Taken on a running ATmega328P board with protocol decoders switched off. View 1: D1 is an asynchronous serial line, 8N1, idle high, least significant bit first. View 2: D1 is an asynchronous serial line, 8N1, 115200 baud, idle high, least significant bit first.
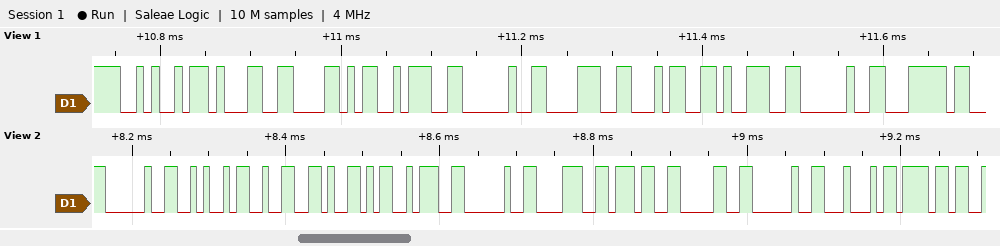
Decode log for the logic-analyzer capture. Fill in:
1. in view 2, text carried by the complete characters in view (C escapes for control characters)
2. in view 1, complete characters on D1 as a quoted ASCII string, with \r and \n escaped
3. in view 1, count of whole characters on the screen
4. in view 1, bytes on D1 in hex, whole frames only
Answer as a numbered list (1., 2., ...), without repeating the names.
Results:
1. " J2Y: 870 Do"
2. "J1X: 849 |"
3. 10
4. 0x4A 0x31 0x58 0x3A 0x20 0x38 0x34 0x39 0x20 0x7C
